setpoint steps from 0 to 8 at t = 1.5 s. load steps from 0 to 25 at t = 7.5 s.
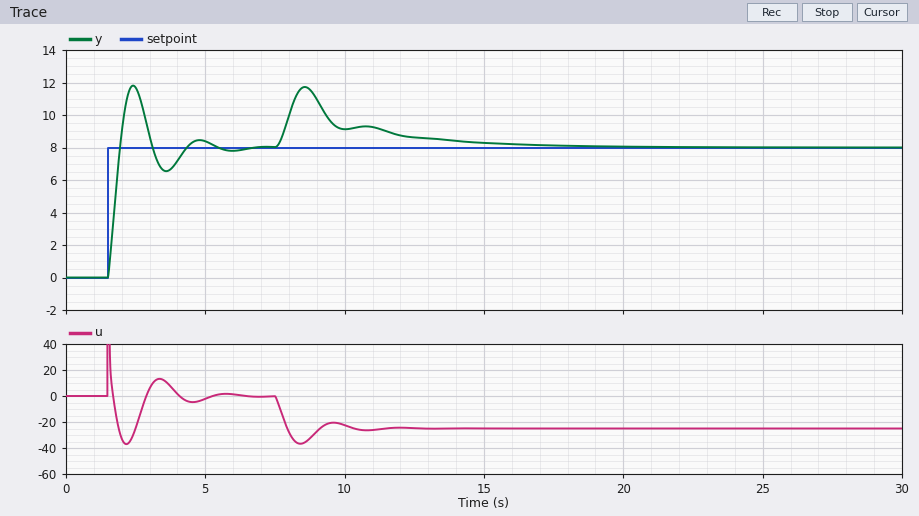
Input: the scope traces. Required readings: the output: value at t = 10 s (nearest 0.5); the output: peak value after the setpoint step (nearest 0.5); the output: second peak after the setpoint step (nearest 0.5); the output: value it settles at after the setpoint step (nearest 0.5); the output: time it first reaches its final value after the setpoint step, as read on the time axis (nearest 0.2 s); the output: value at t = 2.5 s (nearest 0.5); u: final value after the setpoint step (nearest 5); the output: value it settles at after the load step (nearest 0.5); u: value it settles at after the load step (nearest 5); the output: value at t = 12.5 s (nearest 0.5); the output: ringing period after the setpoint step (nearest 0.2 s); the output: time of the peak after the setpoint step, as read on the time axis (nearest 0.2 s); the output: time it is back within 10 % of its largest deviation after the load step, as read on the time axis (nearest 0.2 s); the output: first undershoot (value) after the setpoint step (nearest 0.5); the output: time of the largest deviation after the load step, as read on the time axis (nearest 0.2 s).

9.0
12.0
8.5
8.0
2.0 s
11.5
0
8.0
-25
8.5
2.4 s
2.4 s
14.2 s
6.5
8.6 s
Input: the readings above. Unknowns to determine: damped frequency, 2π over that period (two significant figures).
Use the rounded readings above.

2.6 rad/s
